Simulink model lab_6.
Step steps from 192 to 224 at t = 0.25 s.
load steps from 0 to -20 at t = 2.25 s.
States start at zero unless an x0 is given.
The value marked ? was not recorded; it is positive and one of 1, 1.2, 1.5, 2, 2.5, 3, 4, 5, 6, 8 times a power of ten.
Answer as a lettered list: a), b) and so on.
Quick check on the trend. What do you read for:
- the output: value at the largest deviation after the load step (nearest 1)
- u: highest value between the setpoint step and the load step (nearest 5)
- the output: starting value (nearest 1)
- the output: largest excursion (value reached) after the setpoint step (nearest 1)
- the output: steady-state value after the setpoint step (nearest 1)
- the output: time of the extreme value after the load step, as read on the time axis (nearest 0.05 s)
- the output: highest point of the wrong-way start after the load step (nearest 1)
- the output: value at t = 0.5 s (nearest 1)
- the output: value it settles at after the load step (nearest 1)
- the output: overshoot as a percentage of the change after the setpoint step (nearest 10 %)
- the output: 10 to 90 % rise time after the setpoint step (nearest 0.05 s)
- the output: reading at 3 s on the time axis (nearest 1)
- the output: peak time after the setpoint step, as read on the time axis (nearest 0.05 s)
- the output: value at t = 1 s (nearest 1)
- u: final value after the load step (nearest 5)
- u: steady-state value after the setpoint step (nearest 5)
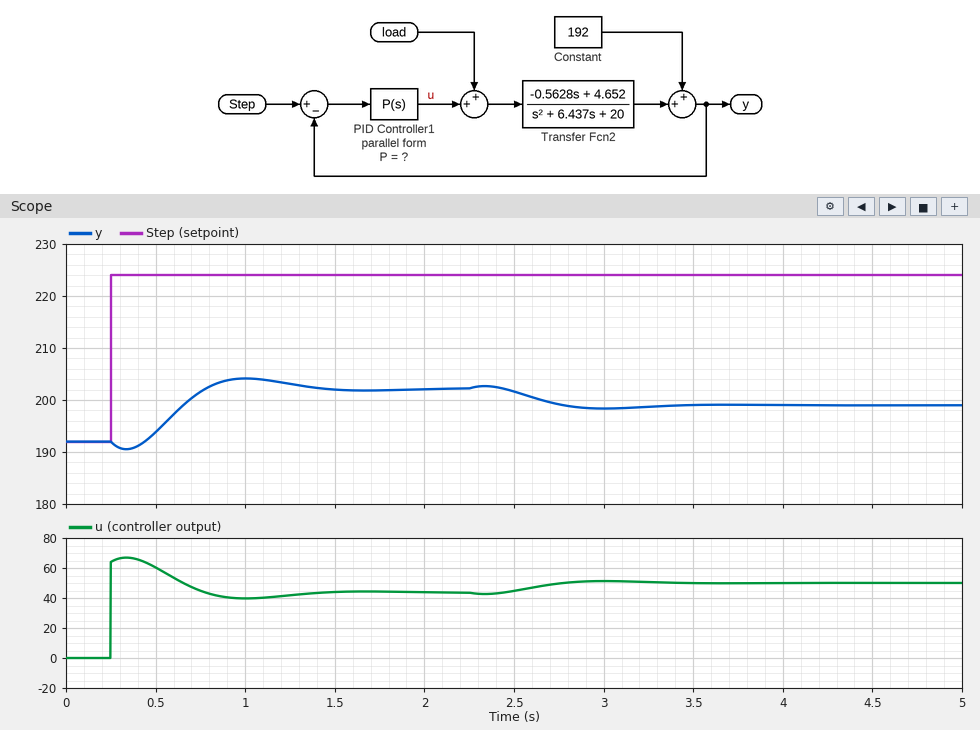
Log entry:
a) 198
b) 65
c) 192
d) 204
e) 202
f) 3.00 s
g) 203
h) 194
i) 199
j) 20 %
k) 0.25 s
l) 198
m) 1.00 s
n) 204
o) 50
p) 45
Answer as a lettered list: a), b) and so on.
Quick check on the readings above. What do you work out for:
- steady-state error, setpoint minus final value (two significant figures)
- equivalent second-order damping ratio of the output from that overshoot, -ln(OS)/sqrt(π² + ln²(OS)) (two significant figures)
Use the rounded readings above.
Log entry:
a) 22
b) 0.46
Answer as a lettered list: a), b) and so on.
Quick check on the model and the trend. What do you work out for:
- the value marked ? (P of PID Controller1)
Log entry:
a) 2
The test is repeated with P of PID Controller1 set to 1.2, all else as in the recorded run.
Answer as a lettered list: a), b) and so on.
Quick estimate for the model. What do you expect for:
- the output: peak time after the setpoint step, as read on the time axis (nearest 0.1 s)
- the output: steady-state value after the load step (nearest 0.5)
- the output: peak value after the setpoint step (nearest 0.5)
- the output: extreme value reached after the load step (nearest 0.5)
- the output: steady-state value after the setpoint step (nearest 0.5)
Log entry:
a) 1.1 s
b) 195.5
c) 200.0
d) 195.0
e) 199.0
